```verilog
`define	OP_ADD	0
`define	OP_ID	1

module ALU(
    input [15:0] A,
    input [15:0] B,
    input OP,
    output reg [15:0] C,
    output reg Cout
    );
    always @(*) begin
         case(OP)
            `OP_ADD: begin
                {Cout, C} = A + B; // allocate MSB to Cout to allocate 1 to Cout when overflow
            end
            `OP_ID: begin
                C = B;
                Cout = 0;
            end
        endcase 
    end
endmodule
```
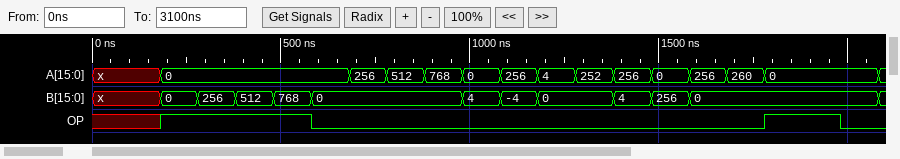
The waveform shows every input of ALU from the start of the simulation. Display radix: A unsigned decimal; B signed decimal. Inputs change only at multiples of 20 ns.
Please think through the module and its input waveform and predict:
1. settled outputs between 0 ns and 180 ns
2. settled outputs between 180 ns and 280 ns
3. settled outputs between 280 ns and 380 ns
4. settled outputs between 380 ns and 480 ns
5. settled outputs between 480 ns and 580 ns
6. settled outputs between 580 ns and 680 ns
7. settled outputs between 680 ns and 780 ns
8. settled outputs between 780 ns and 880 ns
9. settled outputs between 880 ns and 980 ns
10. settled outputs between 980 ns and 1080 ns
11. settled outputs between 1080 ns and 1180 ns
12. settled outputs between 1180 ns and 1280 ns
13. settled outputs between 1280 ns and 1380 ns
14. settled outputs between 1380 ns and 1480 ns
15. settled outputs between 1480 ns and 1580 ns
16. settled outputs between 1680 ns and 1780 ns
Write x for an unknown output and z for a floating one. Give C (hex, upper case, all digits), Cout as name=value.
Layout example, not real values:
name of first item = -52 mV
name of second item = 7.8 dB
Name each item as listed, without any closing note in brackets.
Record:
settled outputs between 0 ns and 180 ns = C=x, Cout=x
settled outputs between 180 ns and 280 ns = C=0000, Cout=0
settled outputs between 280 ns and 380 ns = C=0100, Cout=0
settled outputs between 380 ns and 480 ns = C=0200, Cout=0
settled outputs between 480 ns and 580 ns = C=0300, Cout=0
settled outputs between 580 ns and 680 ns = C=0000, Cout=0
settled outputs between 680 ns and 780 ns = C=0100, Cout=0
settled outputs between 780 ns and 880 ns = C=0200, Cout=0
settled outputs between 880 ns and 980 ns = C=0300, Cout=0
settled outputs between 980 ns and 1080 ns = C=0004, Cout=0
settled outputs between 1080 ns and 1180 ns = C=00FC, Cout=1
settled outputs between 1180 ns and 1280 ns = C=0004, Cout=0
settled outputs between 1280 ns and 1380 ns = C=00FC, Cout=0
settled outputs between 1380 ns and 1480 ns = C=0104, Cout=0
settled outputs between 1480 ns and 1580 ns = C=0100, Cout=0
settled outputs between 1680 ns and 1780 ns = C=0104, Cout=0
